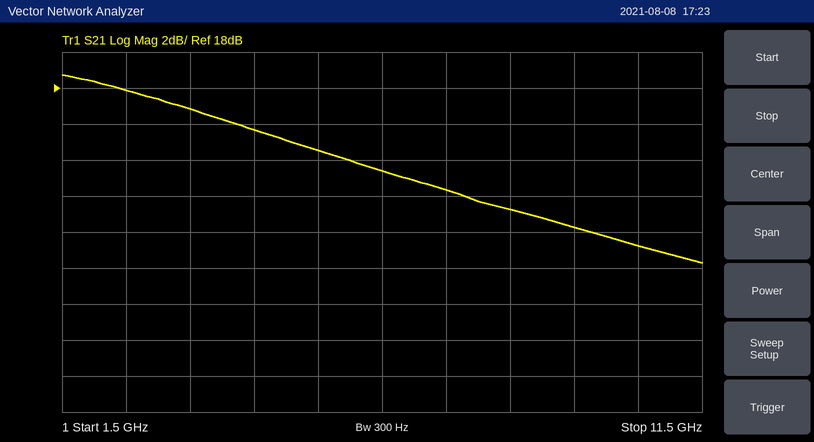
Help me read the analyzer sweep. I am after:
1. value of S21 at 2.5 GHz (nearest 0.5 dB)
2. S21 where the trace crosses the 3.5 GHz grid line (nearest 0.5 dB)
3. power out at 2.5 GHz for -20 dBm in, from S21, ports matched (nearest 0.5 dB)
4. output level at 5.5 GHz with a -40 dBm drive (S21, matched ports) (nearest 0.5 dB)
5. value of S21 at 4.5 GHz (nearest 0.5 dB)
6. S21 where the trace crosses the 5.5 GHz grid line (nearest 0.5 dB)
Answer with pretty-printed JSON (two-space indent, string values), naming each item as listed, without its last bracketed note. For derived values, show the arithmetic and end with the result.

{
  "value of S21 at 2.5 GHz": "18.0 dB",
  "S21 where the trace crosses the 3.5 GHz grid line": "17.0 dB",
  "power out at 2.5 GHz for -20 dBm in, from S21, ports matched": "-20 dBm + (18.0 dB) = -2.0 dBm",
  "output level at 5.5 GHz with a -40 dBm drive (S21, matched ports)": "-40 dBm + (14.5 dB) = -25.5 dBm",
  "value of S21 at 4.5 GHz": "15.5 dB",
  "S21 where the trace crosses the 5.5 GHz grid line": "14.5 dB"
}
